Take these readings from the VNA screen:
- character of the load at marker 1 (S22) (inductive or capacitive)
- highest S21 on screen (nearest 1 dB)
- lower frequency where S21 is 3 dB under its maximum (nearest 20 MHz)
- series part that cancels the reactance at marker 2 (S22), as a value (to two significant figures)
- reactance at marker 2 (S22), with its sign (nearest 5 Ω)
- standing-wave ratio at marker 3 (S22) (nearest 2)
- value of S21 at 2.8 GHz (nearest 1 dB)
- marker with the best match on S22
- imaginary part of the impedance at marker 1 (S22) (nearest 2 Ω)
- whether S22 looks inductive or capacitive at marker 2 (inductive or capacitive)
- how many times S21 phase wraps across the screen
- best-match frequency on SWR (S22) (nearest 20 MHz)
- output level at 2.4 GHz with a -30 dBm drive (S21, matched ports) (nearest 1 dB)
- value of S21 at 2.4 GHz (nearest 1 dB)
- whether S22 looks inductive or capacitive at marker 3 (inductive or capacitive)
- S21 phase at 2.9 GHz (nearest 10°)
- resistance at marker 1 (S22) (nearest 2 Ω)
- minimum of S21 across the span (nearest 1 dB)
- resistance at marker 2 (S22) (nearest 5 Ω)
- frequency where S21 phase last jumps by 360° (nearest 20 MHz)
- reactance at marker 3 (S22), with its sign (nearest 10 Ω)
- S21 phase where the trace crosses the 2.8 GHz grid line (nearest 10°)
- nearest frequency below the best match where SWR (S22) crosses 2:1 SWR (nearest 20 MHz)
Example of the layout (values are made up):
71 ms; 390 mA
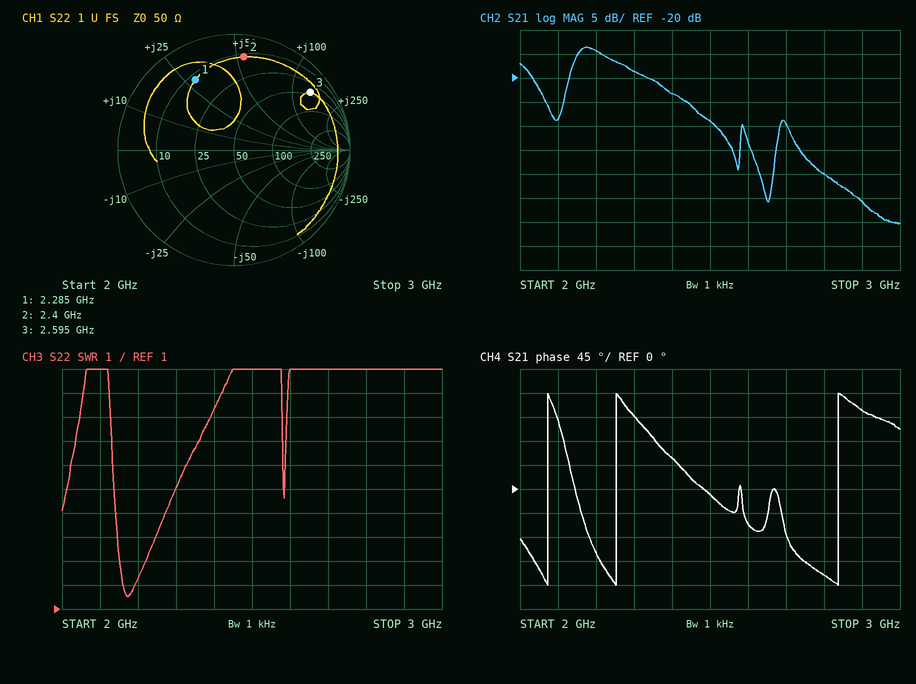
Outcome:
inductive; -14 dB; 2.14 GHz; 1.2 pF; +55 Ω; 10; -40 dB; marker 1; +28 Ω; inductive; 3; 2.18 GHz; -53 dBm; -23 dB; inductive; 150°; 12 Ω; -50 dB; 10 Ω; 2.84 GHz; +140 Ω; -160°; 2.16 GHz
